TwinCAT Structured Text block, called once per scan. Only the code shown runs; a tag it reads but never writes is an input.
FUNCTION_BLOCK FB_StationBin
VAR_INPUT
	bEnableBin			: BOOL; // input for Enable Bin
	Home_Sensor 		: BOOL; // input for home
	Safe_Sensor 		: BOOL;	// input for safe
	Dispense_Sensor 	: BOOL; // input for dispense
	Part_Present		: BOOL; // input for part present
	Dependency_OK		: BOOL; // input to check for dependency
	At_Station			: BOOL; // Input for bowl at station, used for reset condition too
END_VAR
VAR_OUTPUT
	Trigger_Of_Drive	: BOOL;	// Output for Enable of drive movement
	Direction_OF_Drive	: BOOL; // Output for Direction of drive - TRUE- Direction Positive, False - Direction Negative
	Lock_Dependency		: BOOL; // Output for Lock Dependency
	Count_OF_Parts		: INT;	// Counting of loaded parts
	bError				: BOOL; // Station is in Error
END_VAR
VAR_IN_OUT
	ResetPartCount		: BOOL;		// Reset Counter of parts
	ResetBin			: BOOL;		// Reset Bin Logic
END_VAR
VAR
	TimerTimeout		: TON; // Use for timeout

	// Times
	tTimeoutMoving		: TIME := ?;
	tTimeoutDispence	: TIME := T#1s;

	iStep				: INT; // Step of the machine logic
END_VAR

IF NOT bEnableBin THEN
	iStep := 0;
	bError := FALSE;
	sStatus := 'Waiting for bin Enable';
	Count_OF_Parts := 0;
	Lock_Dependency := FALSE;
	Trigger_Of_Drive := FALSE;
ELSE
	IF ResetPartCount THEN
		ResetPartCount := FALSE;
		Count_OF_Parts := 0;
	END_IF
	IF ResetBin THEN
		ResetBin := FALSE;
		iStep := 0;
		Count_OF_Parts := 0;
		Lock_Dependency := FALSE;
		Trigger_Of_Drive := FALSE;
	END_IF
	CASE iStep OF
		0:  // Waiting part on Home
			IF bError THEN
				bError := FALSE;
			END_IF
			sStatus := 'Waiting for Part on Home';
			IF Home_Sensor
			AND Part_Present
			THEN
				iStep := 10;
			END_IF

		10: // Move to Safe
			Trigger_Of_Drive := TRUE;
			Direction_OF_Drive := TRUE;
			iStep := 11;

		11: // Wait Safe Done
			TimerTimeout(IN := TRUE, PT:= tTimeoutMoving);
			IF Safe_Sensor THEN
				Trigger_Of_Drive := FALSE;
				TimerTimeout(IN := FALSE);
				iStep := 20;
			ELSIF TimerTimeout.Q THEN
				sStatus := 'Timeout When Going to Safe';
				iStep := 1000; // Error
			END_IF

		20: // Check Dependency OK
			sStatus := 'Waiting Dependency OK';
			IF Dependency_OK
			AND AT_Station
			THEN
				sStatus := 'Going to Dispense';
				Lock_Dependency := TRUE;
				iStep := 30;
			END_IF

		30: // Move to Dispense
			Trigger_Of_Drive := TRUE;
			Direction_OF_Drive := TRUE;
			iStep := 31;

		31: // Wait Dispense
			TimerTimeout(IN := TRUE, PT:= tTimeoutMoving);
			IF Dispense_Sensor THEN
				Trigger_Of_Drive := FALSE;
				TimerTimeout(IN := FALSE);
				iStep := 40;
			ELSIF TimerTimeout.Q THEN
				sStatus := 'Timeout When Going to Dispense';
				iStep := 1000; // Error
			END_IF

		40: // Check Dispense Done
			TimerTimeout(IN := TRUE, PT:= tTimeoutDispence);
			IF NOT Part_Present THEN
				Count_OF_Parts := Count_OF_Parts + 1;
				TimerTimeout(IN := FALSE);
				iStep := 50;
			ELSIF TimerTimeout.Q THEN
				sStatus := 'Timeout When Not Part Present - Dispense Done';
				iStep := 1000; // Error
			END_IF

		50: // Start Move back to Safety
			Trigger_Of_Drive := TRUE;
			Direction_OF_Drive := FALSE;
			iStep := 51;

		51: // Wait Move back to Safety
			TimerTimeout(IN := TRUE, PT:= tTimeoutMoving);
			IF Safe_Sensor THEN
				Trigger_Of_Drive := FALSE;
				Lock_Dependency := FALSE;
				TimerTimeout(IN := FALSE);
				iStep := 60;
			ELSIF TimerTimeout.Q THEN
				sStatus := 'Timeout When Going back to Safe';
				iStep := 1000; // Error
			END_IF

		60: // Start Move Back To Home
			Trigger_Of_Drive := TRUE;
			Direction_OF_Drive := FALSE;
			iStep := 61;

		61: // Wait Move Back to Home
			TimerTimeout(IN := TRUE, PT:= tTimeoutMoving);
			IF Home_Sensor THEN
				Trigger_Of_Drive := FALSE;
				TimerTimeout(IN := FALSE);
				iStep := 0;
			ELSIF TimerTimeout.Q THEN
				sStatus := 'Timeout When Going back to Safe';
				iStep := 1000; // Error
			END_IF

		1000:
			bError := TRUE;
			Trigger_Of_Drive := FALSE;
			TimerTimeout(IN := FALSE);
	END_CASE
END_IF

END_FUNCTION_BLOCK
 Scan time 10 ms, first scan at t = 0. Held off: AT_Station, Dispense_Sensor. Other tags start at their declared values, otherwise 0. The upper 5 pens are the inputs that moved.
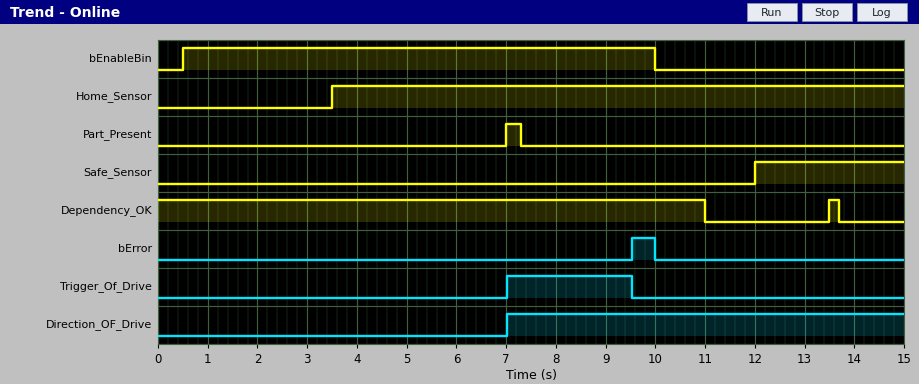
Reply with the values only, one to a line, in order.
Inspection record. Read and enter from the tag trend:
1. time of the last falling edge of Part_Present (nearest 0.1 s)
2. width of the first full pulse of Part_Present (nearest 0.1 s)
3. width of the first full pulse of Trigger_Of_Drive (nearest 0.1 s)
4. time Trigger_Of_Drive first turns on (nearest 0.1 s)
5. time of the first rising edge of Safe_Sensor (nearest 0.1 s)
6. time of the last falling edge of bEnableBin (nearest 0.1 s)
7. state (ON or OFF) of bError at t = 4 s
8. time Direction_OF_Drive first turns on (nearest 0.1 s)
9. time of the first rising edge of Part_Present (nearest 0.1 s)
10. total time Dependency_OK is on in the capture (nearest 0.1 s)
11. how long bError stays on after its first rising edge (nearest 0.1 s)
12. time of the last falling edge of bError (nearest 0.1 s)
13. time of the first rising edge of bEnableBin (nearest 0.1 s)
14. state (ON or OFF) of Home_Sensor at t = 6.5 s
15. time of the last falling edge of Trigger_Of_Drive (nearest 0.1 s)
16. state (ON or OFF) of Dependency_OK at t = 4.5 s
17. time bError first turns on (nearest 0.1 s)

7.3 s
0.3 s
2.5 s
7.0 s
12.0 s
10.0 s
OFF
7.0 s
7.0 s
11.2 s
0.5 s
10.0 s
0.5 s
ON
9.5 s
ON
9.5 s
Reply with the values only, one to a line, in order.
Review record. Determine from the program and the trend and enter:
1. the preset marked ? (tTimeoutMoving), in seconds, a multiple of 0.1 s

2.5 s
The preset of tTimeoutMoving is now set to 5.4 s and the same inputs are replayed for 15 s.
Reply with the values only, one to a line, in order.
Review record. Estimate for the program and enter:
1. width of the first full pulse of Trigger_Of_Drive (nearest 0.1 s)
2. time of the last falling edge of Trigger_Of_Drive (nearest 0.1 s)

3.0 s
10.0 s
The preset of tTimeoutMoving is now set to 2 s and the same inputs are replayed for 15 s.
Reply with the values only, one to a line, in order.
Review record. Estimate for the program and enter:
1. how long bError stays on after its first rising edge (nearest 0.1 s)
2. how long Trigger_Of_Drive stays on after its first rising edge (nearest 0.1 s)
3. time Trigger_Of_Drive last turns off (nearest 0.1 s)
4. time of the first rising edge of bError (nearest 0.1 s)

1.0 s
2.0 s
9.0 s
9.0 s
